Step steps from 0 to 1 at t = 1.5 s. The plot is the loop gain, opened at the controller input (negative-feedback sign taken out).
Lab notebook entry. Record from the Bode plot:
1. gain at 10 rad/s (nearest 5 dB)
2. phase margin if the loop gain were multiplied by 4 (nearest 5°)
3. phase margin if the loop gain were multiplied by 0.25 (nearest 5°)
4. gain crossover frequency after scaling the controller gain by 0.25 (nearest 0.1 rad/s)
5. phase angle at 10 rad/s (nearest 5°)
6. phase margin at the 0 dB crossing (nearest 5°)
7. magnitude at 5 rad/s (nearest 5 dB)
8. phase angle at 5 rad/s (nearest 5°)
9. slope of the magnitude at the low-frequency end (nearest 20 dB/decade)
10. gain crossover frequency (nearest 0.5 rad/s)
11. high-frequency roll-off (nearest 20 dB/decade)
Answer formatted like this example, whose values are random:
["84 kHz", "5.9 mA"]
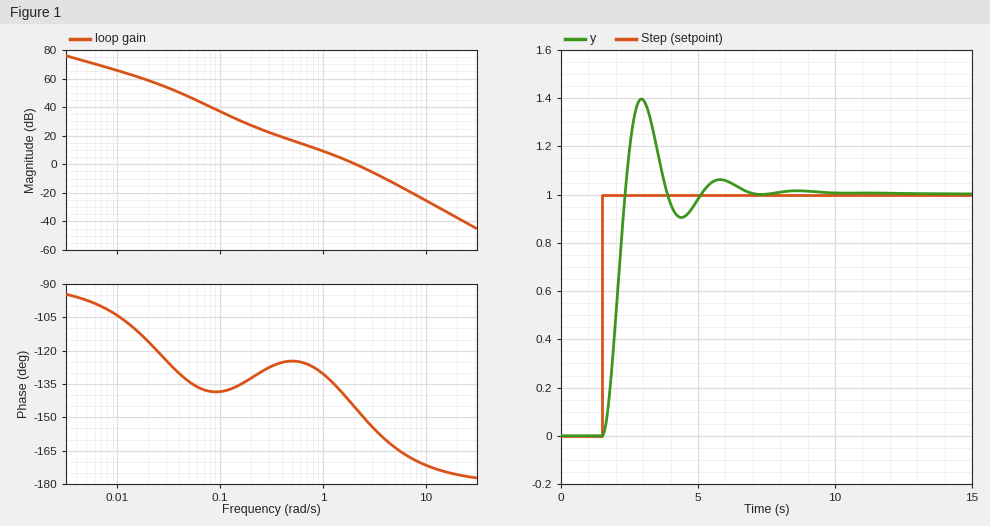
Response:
["-25 dB", "20°", "55°", "0.8 rad/s", "-170°", "35°", "-15 dB", "-165°", "-20 dB/decade", "2.0 rad/s", "-40 dB/decade"]
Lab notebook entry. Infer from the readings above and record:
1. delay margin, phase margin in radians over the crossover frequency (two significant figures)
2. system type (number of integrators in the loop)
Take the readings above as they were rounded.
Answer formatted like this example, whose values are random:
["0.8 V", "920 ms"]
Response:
["0.31 s", "1"]
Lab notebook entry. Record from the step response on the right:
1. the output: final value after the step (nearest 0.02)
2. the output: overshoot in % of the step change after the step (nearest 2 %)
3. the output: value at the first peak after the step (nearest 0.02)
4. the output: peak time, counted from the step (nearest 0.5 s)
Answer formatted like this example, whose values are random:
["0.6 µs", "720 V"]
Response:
["1.00", "40 %", "1.40", "1.5 s"]
